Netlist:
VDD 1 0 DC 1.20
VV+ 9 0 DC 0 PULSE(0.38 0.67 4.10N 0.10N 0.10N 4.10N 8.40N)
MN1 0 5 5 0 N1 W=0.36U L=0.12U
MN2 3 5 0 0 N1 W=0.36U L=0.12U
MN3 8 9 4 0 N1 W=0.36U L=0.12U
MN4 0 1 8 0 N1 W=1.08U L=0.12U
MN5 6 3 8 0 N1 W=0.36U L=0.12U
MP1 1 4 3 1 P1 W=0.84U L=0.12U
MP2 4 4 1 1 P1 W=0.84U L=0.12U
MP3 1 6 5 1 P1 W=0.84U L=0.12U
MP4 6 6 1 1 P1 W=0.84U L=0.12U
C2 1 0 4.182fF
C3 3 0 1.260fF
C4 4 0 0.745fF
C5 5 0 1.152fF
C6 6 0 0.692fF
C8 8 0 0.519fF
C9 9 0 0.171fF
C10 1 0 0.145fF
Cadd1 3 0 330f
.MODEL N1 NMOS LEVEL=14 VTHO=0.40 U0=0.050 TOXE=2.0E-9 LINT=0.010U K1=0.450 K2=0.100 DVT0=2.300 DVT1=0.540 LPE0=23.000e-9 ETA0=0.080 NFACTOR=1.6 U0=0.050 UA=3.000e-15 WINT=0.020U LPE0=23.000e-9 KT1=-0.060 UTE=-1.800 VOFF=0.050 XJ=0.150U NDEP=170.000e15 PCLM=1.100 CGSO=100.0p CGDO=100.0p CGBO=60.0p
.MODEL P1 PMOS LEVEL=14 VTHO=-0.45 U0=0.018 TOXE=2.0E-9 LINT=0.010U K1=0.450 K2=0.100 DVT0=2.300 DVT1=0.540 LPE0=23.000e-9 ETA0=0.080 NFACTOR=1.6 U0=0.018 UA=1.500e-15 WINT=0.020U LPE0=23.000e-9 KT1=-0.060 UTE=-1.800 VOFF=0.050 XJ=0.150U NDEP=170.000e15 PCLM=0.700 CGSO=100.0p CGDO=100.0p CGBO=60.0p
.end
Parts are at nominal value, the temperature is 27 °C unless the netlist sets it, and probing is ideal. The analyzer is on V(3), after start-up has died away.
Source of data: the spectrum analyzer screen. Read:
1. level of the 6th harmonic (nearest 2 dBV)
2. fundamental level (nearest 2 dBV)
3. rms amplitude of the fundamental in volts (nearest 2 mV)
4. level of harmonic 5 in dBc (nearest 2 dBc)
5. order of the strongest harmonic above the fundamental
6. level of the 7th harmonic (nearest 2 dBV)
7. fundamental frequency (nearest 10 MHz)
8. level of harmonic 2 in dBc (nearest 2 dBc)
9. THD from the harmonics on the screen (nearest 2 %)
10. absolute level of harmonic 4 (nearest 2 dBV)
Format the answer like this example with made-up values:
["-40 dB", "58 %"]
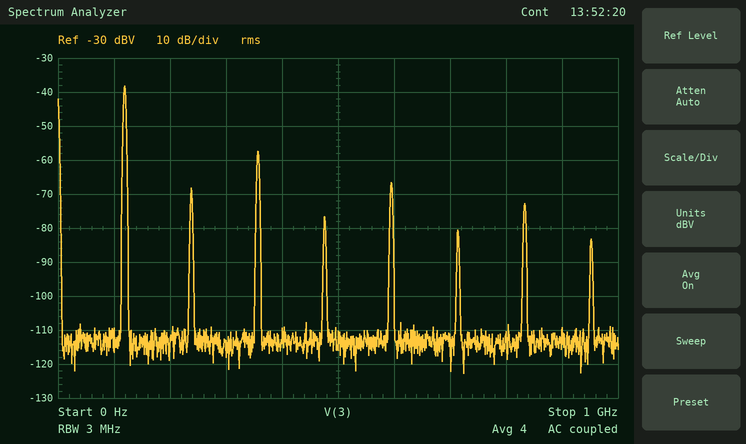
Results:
["-80 dBV", "-38 dBV", "12 mV", "-28 dBc", "3", "-72 dBV", "120 MHz", "-30 dBc", "12 %", "-76 dBV"]
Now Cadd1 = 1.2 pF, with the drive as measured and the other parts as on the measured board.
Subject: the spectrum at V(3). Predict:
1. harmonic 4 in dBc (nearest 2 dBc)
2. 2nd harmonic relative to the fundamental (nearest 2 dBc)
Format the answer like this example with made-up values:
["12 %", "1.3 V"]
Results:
["-40 dBc", "-34 dBc"]
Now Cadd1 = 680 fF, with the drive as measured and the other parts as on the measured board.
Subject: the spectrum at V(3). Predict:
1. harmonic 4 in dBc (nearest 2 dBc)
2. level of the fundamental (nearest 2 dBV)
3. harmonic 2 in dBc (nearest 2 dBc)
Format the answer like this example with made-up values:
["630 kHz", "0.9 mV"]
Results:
["-40 dBc", "-44 dBV", "-34 dBc"]
